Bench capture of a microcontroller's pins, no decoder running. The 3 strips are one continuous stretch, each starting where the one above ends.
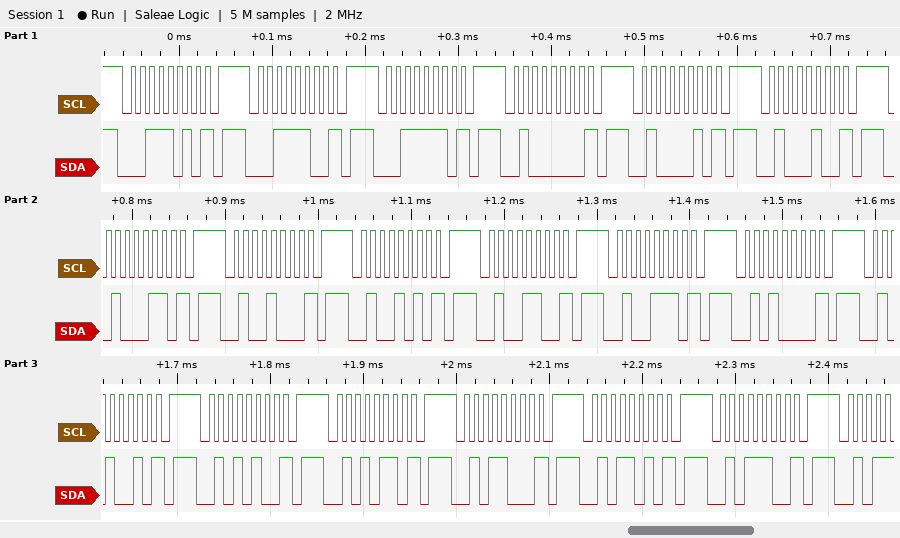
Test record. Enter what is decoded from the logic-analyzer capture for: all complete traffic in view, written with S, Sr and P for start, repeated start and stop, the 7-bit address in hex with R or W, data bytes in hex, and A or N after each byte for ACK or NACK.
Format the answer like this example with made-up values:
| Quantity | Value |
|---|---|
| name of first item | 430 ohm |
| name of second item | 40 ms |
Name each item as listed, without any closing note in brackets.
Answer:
| Quantity | Value |
|---|---|
| all complete traffic in view, written with S, Sr and P for start, repeated start and stop, the 7-bit address in hex with R or W, data bytes in hex, and A or N after each byte for ACK or NACK | S 1DW N P S 1EW N P S 1FW N P S 20W N P S 21W N P S 22W N P S 23W N P S 24W N P S 25W N P S 26W N P S 27W N P S 28W N P S 29W N P S 2AW N P S 2BW N P S 2CW N P S 2DW N P S 2EW N P |
